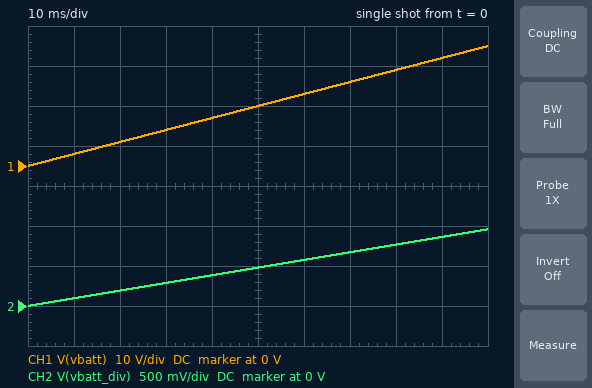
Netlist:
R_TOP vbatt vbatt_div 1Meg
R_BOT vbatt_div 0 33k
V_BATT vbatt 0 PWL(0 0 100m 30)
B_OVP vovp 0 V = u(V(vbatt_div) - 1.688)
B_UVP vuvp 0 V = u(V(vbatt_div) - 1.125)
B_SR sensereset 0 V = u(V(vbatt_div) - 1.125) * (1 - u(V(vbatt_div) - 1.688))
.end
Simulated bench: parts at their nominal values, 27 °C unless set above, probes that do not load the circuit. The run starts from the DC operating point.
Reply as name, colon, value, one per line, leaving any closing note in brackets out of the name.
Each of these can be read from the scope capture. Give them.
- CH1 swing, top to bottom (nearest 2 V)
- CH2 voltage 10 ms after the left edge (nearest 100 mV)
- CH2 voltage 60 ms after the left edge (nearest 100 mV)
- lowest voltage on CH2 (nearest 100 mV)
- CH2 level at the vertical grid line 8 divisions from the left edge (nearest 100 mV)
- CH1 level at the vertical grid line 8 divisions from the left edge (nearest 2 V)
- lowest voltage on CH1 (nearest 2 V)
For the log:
CH1 swing, top to bottom: 30 V
CH2 voltage 10 ms after the left edge: 100 mV
CH2 voltage 60 ms after the left edge: 600 mV
lowest voltage on CH2: 0 V
CH2 level at the vertical grid line 8 divisions from the left edge: 800 mV
CH1 level at the vertical grid line 8 divisions from the left edge: 24 V
lowest voltage on CH1: 0 V
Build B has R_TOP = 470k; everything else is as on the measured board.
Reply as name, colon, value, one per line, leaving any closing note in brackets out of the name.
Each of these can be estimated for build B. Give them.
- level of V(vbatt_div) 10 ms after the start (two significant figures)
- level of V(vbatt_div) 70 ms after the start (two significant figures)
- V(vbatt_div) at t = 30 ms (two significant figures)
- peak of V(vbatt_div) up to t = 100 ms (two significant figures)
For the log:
level of V(vbatt_div) 10 ms after the start: 200 mV
level of V(vbatt_div) 70 ms after the start: 1.4 V
V(vbatt_div) at t = 30 ms: 590 mV
peak of V(vbatt_div) up to t = 100 ms: 2.0 V
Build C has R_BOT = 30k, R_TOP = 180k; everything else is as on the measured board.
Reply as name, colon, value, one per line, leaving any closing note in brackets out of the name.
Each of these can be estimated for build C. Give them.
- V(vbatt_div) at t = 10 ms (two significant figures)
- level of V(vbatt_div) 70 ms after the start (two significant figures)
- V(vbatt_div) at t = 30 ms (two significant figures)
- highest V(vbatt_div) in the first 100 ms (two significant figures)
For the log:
V(vbatt_div) at t = 10 ms: 430 mV
level of V(vbatt_div) 70 ms after the start: 3.0 V
V(vbatt_div) at t = 30 ms: 1.3 V
highest V(vbatt_div) in the first 100 ms: 4.3 V
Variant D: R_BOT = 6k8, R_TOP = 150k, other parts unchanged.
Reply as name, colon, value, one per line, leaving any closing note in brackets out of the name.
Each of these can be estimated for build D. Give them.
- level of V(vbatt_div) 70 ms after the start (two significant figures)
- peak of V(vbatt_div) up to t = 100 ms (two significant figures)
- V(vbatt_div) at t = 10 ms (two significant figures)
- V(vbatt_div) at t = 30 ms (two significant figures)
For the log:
level of V(vbatt_div) 70 ms after the start: 910 mV
peak of V(vbatt_div) up to t = 100 ms: 1.3 V
V(vbatt_div) at t = 10 ms: 130 mV
V(vbatt_div) at t = 30 ms: 390 mV
